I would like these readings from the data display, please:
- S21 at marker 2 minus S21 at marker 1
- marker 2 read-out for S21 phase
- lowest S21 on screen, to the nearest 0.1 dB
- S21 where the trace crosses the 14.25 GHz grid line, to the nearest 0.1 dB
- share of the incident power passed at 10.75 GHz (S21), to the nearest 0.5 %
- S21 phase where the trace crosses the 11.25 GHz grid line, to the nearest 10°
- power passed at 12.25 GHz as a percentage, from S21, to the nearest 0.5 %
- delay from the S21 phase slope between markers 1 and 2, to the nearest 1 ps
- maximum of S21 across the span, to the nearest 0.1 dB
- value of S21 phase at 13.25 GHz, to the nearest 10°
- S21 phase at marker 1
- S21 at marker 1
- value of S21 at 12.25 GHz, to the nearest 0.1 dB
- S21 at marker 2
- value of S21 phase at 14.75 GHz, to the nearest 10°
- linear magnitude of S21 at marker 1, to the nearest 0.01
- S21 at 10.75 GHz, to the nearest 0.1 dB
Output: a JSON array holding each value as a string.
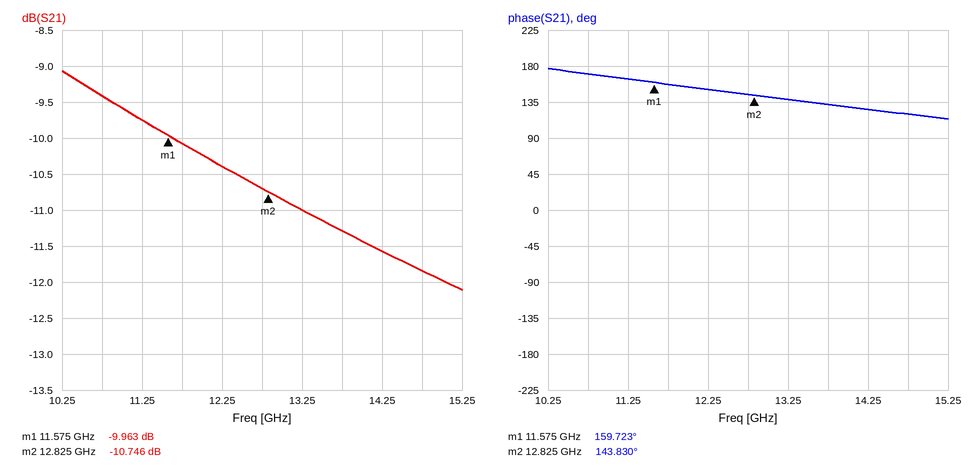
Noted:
["-0.783 dB", "143.830°", "-12.1 dB", "-11.6 dB", "11.5 %", "160°", "9.0 %", "35 ps", "-9.1 dB", "140°", "159.723°", "-9.963 dB", "-10.4 dB", "-10.746 dB", "120°", "0.32", "-9.4 dB"]
